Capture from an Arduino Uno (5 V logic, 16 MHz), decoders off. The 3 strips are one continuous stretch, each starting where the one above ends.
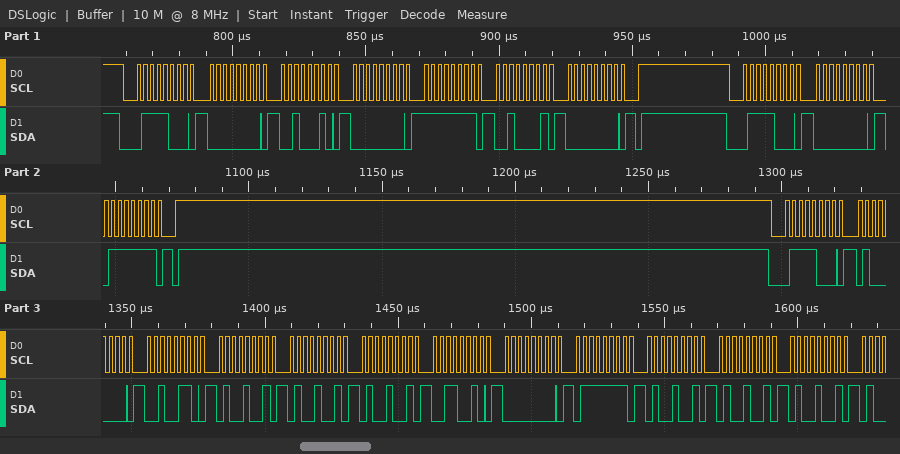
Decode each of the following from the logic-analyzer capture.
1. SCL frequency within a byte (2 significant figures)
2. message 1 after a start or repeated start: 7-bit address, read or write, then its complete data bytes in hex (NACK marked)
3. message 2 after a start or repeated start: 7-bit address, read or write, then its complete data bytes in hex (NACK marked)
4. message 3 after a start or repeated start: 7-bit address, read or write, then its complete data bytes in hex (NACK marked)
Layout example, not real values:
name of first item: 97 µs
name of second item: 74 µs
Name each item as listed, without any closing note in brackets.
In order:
SCL frequency within a byte: 400 kHz
message 1 after a start or repeated start: 7-bit address, read or write, then its complete data bytes in hex: 0x3C write: 00 22 00 FF 21 00
message 2 after a start or repeated start: 7-bit address, read or write, then its complete data bytes in hex: 0x3C write: 00 7F
message 3 after a start or repeated start: 7-bit address, read or write, then its complete data bytes in hex: 0x3C write: 40 26 49 49 49 32 00 7F 49 49 49
